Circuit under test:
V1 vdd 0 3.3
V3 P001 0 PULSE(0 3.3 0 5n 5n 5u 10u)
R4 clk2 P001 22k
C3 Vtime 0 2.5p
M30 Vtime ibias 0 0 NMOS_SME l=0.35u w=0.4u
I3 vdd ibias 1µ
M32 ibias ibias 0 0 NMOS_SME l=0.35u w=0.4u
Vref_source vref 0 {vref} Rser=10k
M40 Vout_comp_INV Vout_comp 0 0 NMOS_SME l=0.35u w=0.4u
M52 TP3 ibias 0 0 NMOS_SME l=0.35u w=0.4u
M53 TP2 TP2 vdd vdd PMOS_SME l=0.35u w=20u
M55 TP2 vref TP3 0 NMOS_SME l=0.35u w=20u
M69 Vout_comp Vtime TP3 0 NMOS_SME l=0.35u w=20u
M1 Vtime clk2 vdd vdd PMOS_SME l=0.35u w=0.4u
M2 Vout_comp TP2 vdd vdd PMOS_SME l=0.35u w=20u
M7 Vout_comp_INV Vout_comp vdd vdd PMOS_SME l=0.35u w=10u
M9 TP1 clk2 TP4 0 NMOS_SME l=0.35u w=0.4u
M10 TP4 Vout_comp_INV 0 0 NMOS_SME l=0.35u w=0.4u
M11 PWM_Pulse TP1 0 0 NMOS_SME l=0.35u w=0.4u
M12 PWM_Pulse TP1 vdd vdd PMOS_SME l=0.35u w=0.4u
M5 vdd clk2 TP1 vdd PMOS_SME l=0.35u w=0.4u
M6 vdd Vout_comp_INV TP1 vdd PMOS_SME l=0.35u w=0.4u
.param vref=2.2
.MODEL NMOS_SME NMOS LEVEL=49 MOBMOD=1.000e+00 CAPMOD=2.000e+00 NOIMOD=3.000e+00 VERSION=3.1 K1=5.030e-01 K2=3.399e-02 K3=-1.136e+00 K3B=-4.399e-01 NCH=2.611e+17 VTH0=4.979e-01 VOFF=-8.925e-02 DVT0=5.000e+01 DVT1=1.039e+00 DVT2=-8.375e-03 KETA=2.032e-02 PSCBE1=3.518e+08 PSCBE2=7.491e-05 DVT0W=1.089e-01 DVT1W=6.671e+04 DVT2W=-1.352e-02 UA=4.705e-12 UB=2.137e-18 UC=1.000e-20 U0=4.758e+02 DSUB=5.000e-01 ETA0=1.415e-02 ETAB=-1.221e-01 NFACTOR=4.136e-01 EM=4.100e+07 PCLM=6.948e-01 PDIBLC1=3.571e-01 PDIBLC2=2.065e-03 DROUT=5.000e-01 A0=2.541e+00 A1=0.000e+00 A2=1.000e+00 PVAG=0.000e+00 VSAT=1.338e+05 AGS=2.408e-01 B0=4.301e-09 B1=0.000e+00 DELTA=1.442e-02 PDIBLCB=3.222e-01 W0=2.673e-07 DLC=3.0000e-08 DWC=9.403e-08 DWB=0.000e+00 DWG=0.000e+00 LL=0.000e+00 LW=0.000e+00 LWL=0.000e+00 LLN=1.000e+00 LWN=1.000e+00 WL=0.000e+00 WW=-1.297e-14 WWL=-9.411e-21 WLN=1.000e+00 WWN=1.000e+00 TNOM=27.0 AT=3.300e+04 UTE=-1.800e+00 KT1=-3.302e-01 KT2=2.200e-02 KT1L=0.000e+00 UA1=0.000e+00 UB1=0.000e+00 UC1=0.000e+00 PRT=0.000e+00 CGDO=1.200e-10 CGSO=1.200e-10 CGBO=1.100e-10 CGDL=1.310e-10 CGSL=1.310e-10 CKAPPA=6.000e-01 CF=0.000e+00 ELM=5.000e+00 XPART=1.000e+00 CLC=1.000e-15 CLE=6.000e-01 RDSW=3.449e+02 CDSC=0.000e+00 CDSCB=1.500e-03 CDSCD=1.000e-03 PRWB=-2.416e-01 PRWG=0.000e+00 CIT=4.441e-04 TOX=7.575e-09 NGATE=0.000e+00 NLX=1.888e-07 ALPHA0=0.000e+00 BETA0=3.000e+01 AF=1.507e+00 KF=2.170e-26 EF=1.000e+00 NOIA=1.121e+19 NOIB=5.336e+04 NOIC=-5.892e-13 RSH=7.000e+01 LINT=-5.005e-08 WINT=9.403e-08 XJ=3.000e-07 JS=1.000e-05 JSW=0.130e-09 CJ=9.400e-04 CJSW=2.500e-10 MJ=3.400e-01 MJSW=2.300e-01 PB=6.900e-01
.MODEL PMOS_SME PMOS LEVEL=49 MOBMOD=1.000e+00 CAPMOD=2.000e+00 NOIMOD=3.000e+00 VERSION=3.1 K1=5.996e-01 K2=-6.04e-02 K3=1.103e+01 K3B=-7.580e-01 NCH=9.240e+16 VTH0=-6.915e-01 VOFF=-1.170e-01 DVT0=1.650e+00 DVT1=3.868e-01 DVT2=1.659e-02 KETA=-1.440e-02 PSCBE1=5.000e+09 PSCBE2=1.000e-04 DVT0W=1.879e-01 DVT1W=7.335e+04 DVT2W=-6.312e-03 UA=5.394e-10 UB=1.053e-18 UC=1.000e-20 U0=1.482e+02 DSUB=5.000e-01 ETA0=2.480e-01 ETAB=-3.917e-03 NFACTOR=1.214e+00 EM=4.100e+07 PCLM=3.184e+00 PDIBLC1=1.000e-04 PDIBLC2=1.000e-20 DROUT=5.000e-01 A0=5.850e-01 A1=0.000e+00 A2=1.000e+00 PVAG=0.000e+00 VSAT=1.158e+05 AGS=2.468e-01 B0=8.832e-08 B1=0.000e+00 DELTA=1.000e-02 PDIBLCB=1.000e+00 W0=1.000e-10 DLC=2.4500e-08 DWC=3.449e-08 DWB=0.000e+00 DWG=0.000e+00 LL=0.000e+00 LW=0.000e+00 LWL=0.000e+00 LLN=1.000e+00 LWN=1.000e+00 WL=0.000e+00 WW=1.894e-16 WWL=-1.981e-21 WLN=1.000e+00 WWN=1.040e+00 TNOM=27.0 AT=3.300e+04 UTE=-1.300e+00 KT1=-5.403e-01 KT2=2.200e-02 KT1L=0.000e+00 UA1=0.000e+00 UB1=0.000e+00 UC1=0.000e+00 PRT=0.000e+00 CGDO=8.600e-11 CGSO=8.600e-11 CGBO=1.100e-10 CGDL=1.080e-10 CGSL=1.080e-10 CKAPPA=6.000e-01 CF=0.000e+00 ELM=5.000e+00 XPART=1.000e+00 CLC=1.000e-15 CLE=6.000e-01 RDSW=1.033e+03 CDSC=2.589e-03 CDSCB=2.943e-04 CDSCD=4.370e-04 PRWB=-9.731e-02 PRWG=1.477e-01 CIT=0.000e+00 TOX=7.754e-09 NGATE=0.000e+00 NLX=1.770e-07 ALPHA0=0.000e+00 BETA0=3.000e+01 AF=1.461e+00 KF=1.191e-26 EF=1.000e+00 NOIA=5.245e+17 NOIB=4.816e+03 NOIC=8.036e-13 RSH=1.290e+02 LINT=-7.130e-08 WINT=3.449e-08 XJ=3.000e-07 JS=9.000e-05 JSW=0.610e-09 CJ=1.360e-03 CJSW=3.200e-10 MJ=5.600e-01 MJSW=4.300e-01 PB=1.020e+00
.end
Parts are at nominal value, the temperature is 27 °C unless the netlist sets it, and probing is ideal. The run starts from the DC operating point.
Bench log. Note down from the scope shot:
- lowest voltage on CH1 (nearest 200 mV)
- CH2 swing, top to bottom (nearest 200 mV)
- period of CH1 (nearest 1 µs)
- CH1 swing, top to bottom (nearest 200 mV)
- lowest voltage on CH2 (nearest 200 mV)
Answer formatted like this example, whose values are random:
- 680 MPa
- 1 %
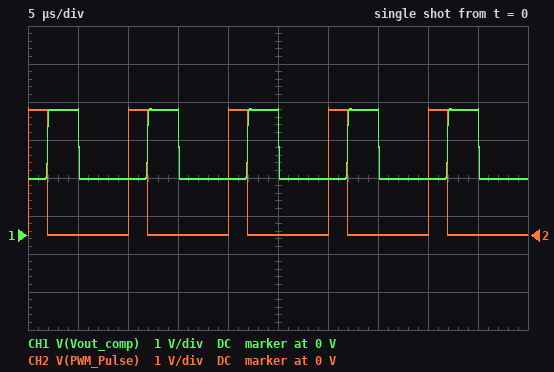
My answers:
- 1.4 V
- 3.4 V
- 10 µs
- 1.8 V
- 0 V
